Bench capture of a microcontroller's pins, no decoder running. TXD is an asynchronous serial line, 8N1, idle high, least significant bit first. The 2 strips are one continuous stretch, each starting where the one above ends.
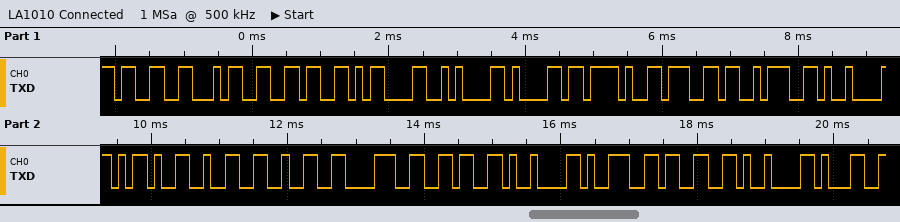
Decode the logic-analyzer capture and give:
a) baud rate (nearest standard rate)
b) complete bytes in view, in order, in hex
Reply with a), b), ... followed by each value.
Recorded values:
a) 9600 baud
b) 33 34 36 0D 0A 61 2F 67 3A 09 2D 32 32 38 36 09 39 33 09 31
